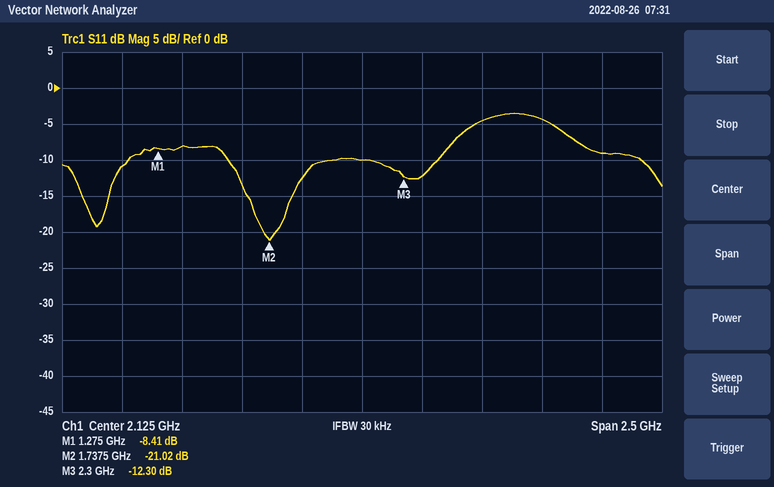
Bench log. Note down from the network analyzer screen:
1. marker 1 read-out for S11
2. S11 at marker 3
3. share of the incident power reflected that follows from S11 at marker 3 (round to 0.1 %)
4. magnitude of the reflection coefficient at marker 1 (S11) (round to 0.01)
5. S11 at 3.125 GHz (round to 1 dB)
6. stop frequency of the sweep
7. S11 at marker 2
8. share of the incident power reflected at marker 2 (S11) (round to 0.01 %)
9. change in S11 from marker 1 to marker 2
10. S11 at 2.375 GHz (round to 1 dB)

-8.41 dB
-12.30 dB
5.9 %
0.38
-9 dB
3.375 GHz
-21.02 dB
0.79 %
-12.61 dB
-12 dB
